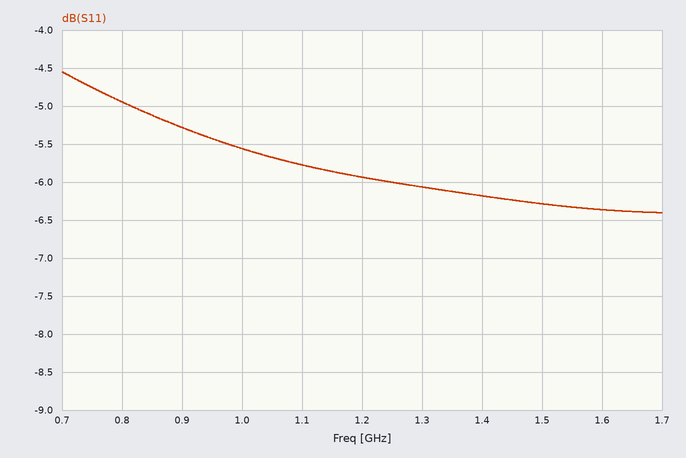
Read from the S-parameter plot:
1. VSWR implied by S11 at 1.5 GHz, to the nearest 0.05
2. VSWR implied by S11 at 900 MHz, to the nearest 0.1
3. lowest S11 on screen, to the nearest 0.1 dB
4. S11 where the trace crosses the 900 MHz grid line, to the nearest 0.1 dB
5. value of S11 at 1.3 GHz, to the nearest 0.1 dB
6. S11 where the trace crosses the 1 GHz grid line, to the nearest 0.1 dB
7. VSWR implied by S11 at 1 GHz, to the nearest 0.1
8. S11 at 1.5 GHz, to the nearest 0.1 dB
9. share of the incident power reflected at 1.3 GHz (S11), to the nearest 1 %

2.90
3.4
-6.4 dB
-5.3 dB
-6.1 dB
-5.6 dB
3.2
-6.3 dB
25 %
